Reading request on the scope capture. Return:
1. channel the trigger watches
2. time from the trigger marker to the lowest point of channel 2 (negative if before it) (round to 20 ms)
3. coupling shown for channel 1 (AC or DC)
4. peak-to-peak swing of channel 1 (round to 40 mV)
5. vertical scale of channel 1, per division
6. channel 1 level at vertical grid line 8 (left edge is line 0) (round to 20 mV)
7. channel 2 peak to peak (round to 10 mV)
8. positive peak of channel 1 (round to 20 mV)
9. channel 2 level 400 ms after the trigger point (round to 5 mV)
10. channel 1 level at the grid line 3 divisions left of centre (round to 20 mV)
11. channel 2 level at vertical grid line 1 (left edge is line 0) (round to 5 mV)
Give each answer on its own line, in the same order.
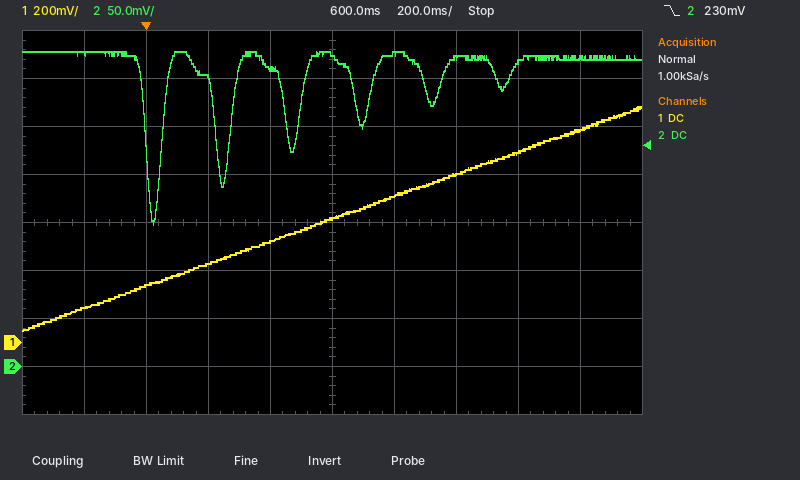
channel 2
+20 ms
DC
920 mV
200 mV
800 mV
180 mV
980 mV
310 mV
240 mV
325 mV
